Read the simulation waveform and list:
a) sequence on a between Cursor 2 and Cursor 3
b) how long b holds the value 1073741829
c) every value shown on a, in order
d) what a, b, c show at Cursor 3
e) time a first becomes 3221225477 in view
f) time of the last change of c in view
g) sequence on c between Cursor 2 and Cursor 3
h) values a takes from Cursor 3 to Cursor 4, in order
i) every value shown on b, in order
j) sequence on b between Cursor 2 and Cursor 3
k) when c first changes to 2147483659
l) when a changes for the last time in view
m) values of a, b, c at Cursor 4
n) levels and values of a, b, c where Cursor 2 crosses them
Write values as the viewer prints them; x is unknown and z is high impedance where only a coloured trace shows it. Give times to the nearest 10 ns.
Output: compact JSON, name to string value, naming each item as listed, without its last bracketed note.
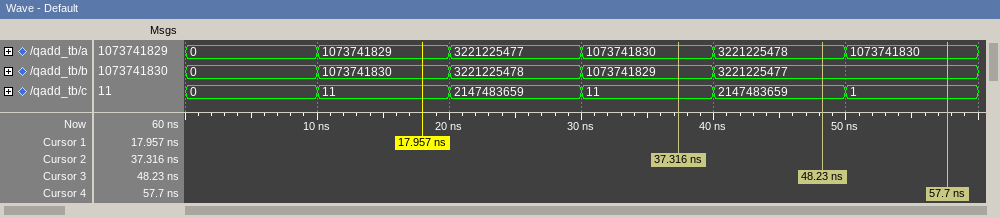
{"sequence on a between Cursor 2 and Cursor 3": "1073741830, 3221225478", "how long b holds the value 1073741829": "10 ns", "every value shown on a, in order": "0, 1073741829, 3221225477, 1073741830, 3221225478, 1073741830", "what a, b, c show at Cursor 3": "a=3221225478, b=3221225477, c=2147483659", "time a first becomes 3221225477 in view": "20 ns", "time of the last change of c in view": "50 ns", "sequence on c between Cursor 2 and Cursor 3": "11, 2147483659", "values a takes from Cursor 3 to Cursor 4, in order": "3221225478, 1073741830", "every value shown on b, in order": "0, 1073741830, 3221225478, 1073741829, 3221225477", "sequence on b between Cursor 2 and Cursor 3": "1073741829, 3221225477", "when c first changes to 2147483659": "20 ns", "when a changes for the last time in view": "50 ns", "values of a, b, c at Cursor 4": "a=1073741830, b=3221225477, c=1", "levels and values of a, b, c where Cursor 2 crosses them": "a=1073741830, b=1073741829, c=11"}
